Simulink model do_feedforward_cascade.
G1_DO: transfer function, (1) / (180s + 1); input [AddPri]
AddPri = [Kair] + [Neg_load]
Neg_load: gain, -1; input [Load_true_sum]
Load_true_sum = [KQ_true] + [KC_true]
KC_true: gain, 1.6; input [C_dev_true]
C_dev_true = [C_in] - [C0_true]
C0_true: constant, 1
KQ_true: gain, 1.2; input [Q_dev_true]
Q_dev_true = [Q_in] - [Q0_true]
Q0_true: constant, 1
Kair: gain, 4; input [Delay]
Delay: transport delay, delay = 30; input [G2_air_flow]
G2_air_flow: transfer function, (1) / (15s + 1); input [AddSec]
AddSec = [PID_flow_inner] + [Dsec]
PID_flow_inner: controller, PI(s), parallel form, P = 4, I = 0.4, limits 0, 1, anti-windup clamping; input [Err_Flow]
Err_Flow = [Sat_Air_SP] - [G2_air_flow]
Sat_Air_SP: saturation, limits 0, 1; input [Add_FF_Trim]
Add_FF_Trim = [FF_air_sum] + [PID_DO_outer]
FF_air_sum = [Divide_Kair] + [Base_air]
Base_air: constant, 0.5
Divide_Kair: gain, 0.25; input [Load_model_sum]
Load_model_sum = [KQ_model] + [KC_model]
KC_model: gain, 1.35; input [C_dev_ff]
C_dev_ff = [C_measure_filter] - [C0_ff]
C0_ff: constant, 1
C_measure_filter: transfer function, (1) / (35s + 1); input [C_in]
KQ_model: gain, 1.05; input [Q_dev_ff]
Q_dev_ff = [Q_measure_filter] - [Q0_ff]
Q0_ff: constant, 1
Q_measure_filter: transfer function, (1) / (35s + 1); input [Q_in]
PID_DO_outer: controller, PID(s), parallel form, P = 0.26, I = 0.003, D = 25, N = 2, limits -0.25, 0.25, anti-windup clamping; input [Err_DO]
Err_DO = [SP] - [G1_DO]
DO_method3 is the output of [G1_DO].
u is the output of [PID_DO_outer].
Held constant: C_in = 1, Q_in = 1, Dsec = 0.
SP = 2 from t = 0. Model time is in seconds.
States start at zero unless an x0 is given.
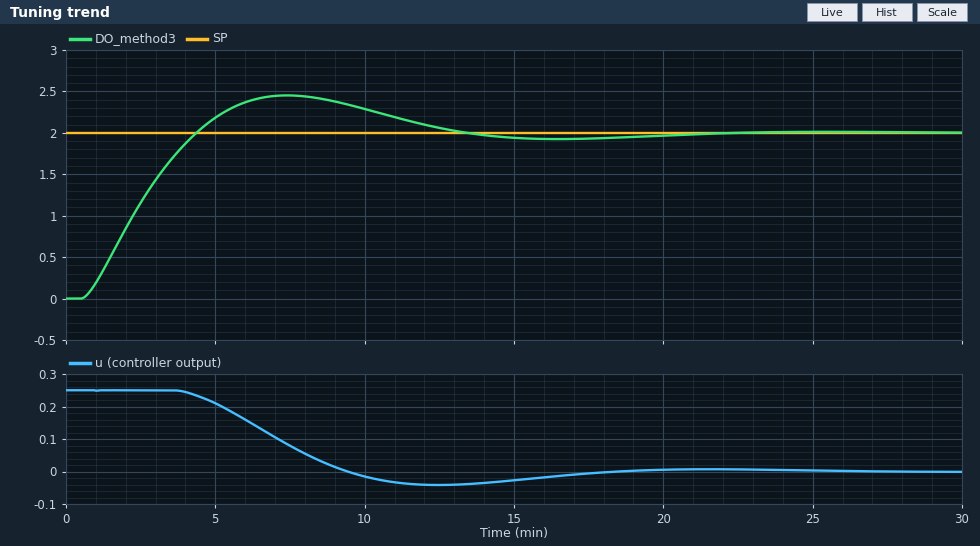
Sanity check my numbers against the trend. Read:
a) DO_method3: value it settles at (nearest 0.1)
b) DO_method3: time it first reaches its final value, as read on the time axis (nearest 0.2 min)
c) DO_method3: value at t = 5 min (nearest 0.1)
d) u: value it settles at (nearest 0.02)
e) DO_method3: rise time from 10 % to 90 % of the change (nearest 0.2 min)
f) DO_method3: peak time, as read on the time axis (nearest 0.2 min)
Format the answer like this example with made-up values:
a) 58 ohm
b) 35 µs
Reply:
a) 2.0
b) 4.4 min
c) 2.2
d) 0.00
e) 2.8 min
f) 7.4 min
